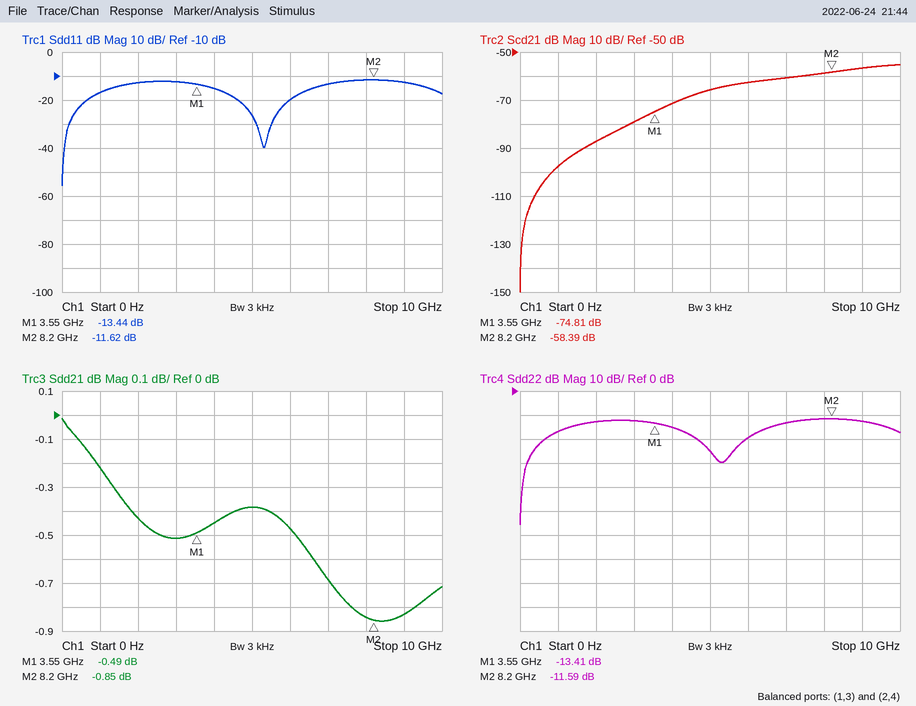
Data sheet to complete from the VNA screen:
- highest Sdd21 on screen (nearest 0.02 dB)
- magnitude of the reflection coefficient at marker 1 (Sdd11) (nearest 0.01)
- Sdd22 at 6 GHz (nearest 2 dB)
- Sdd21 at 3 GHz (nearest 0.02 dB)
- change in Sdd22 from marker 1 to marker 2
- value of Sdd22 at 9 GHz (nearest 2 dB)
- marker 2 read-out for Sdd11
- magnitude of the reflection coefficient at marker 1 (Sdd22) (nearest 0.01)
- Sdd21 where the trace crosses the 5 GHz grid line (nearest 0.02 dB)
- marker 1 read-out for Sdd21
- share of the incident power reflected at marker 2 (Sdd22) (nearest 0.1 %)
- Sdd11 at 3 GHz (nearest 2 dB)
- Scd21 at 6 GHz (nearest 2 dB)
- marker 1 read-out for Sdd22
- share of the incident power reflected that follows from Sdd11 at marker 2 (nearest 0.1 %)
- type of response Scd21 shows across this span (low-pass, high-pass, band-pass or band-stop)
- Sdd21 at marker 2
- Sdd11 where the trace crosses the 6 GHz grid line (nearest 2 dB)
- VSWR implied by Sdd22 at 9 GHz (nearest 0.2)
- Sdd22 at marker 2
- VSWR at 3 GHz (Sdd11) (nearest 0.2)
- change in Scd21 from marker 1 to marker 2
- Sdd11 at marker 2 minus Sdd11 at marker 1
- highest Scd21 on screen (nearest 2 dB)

-0.02 dB
0.21
-20 dB
-0.52 dB
1.82 dB
-12 dB
-11.62 dB
0.21
-0.38 dB
-0.49 dB
6.9 %
-12 dB
-62 dB
-13.41 dB
6.9 %
high-pass
-0.85 dB
-20 dB
1.6
-11.59 dB
1.6
16.42 dB
1.82 dB
-56 dB
